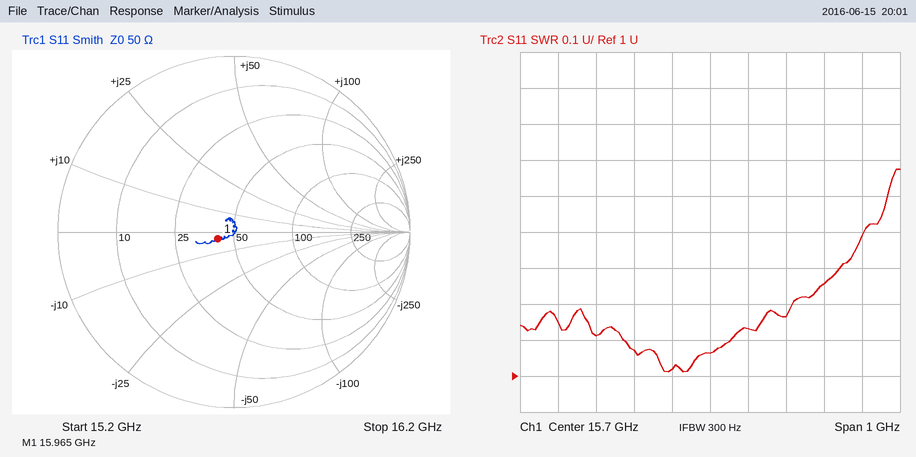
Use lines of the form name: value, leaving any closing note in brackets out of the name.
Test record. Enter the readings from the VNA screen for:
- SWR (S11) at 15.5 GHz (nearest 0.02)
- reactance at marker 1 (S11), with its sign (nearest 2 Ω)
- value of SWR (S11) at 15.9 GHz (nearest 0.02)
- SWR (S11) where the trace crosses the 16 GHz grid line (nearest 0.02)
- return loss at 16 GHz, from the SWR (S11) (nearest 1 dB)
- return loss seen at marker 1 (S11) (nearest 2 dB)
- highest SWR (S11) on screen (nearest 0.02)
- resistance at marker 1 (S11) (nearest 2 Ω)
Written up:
SWR (S11) at 15.5 GHz: 1.08
reactance at marker 1 (S11), with its sign: -4 Ω
value of SWR (S11) at 15.9 GHz: 1.16
SWR (S11) where the trace crosses the 16 GHz grid line: 1.26
return loss at 16 GHz, from the SWR (S11): 19 dB
return loss seen at marker 1 (S11): 20 dB
highest SWR (S11) on screen: 1.58
resistance at marker 1 (S11): 42 Ω
